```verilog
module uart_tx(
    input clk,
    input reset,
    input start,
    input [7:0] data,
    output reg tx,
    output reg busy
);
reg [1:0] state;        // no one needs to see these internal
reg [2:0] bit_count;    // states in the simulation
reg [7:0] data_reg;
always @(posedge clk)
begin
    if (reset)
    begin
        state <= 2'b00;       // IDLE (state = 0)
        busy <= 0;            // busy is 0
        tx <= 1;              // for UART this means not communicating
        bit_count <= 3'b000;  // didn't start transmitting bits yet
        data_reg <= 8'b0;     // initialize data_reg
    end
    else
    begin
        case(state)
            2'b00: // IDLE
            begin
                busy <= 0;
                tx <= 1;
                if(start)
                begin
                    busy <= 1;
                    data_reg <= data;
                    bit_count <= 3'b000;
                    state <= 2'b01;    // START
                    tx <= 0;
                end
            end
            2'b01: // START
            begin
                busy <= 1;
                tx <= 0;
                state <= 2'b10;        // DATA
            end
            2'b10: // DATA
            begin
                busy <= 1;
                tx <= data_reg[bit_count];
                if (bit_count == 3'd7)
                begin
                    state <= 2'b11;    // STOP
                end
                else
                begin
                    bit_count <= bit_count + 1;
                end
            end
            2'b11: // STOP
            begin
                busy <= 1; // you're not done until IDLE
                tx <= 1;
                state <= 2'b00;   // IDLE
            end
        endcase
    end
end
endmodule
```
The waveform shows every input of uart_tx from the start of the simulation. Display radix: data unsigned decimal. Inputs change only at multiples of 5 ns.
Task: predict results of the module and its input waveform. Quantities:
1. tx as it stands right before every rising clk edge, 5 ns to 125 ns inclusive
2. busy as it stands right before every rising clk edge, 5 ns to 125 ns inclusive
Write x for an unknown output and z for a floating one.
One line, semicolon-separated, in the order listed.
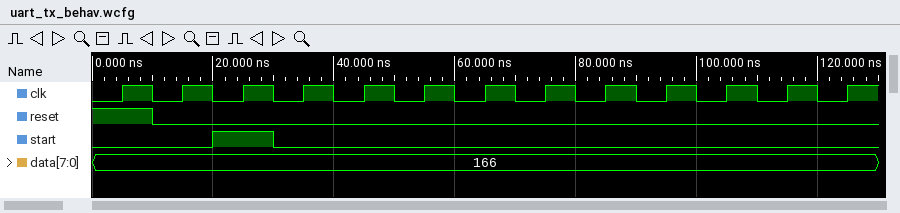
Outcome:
x 1 1 0 0 0 1 1 0 0 1 0 1; x 0 0 1 1 1 1 1 1 1 1 1 1
